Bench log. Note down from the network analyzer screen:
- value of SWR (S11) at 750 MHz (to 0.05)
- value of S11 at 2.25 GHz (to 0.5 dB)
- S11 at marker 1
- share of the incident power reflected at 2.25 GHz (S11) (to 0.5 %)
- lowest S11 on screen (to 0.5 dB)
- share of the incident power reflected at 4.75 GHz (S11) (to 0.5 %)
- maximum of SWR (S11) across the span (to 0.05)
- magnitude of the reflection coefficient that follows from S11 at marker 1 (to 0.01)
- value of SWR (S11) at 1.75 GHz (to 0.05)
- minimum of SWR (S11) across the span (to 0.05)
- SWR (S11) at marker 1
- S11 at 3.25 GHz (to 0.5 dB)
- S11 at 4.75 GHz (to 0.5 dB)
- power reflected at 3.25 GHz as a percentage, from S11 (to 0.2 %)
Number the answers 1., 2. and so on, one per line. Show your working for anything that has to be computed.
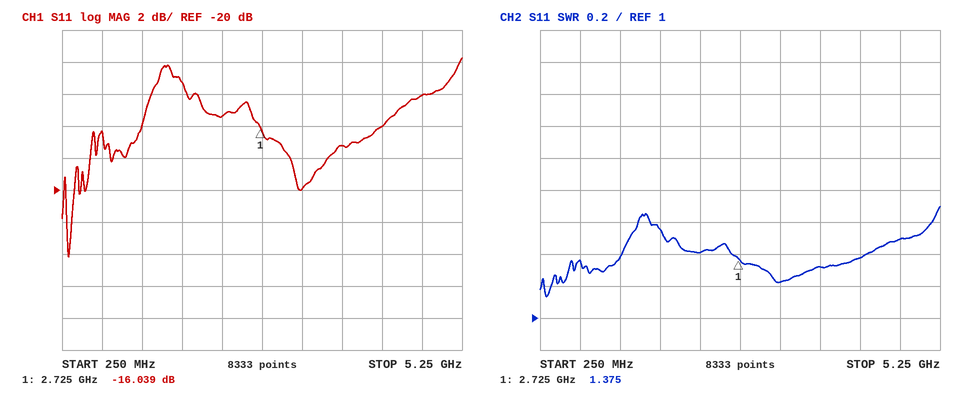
1. 1.35
2. -15.5 dB
3. -16.039 dB
4. 10^(-15.5/10) ≈ 2.82 %, so 3.0 % to the nearest 0.5 %
5. -24.0 dB
6. 10^(-14/10) ≈ 4.0 %
7. 1.70
8. 10^(-16.039/20) ≈ 0.16
9. 1.55
10. 1.15
11. 1.375
12. -20.0 dB
13. -14.0 dB
14. 10^(-20/10) ≈ 1.0 %
